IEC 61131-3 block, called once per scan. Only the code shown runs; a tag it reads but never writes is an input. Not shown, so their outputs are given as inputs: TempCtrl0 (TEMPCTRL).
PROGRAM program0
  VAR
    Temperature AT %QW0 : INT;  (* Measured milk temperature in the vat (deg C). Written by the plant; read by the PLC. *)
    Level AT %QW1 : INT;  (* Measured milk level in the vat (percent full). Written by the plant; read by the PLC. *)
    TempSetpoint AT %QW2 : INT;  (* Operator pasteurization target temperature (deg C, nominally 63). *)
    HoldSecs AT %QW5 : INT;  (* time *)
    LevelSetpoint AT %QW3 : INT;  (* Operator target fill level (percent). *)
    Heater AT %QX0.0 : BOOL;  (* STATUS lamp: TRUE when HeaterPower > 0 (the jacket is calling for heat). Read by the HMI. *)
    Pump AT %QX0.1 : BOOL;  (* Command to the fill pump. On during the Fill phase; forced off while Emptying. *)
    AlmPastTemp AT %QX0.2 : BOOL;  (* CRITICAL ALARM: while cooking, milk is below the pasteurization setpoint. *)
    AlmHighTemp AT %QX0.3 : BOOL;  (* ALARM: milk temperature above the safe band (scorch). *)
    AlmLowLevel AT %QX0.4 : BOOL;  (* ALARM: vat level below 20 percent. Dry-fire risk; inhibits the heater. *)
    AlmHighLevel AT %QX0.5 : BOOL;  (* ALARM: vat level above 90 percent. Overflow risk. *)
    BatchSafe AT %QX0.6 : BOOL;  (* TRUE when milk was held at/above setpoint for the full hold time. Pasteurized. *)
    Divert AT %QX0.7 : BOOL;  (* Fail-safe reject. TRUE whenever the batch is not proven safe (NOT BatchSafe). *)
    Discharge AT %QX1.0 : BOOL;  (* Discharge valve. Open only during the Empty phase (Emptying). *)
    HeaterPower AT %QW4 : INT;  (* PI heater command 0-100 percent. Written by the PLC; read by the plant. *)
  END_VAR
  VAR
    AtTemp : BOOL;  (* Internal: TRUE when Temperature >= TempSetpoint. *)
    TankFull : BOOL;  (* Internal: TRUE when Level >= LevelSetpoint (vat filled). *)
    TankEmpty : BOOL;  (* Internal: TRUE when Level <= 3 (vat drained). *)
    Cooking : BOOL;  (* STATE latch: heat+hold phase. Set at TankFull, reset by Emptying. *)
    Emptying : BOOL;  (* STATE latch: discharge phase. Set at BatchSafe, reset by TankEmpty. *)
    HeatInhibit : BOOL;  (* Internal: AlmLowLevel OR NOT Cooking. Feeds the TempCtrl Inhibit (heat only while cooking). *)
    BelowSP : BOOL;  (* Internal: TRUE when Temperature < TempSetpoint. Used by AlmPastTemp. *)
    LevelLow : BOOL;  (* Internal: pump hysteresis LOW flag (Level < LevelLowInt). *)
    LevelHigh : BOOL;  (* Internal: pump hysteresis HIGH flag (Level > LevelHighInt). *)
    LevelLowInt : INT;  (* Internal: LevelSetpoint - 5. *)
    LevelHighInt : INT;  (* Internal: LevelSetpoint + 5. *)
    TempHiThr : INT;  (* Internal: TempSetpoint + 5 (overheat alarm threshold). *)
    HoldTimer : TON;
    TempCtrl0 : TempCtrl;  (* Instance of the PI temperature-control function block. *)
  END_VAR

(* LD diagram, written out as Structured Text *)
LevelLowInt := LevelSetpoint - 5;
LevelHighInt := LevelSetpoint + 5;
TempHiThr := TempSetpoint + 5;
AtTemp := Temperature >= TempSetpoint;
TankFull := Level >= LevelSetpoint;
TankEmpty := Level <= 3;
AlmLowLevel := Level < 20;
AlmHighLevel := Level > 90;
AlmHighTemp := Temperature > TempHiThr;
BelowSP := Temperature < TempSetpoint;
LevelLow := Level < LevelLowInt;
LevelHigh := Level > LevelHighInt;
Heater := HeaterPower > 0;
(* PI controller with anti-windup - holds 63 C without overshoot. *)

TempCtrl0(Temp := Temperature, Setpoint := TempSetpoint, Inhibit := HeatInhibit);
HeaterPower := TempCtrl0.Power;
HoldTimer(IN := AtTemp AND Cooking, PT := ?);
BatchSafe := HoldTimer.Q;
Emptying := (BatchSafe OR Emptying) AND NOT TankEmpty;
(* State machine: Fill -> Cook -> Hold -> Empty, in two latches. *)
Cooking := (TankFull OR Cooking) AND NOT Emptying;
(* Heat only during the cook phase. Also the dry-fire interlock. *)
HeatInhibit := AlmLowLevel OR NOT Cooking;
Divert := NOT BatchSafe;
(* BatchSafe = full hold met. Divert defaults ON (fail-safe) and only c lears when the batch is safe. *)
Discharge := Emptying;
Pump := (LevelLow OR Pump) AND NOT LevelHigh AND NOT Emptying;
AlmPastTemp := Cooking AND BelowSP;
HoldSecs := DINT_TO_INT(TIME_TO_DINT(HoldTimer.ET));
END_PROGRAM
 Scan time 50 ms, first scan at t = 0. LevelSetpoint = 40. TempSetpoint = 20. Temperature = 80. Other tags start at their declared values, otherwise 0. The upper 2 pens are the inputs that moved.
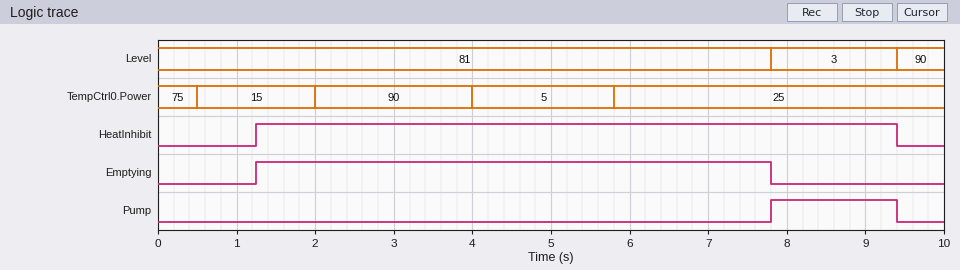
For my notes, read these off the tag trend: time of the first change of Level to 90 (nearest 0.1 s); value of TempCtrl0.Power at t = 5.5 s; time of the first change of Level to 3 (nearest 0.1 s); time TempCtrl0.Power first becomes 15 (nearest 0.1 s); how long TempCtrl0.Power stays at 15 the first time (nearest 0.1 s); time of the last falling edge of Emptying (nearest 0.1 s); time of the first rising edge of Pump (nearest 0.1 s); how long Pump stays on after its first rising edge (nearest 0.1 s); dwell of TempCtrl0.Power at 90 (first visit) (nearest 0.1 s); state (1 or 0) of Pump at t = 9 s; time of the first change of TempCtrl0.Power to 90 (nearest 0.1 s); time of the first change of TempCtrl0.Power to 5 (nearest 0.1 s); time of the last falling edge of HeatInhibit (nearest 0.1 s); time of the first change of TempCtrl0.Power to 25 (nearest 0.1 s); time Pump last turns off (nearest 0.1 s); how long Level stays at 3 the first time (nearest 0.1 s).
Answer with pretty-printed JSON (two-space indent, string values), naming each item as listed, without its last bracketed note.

{
  "time of the first change of Level to 90": "9.4 s",
  "value of TempCtrl0.Power at t = 5.5 s": "5",
  "time of the first change of Level to 3": "7.8 s",
  "time TempCtrl0.Power first becomes 15": "0.5 s",
  "how long TempCtrl0.Power stays at 15 the first time": "1.5 s",
  "time of the last falling edge of Emptying": "7.8 s",
  "time of the first rising edge of Pump": "7.8 s",
  "how long Pump stays on after its first rising edge": "1.6 s",
  "dwell of TempCtrl0.Power at 90 (first visit)": "2.0 s",
  "state (1 or 0) of Pump at t = 9 s": "1",
  "time of the first change of TempCtrl0.Power to 90": "2.0 s",
  "time of the first change of TempCtrl0.Power to 5": "4.0 s",
  "time of the last falling edge of HeatInhibit": "9.4 s",
  "time of the first change of TempCtrl0.Power to 25": "5.8 s",
  "time Pump last turns off": "9.4 s",
  "how long Level stays at 3 the first time": "1.6 s"
}
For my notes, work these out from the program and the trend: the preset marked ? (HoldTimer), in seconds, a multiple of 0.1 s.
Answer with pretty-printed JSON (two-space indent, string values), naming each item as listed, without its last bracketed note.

{
  "the preset marked ? (HoldTimer), in seconds, a multiple of 0.1 s": "1.2 s"
}
